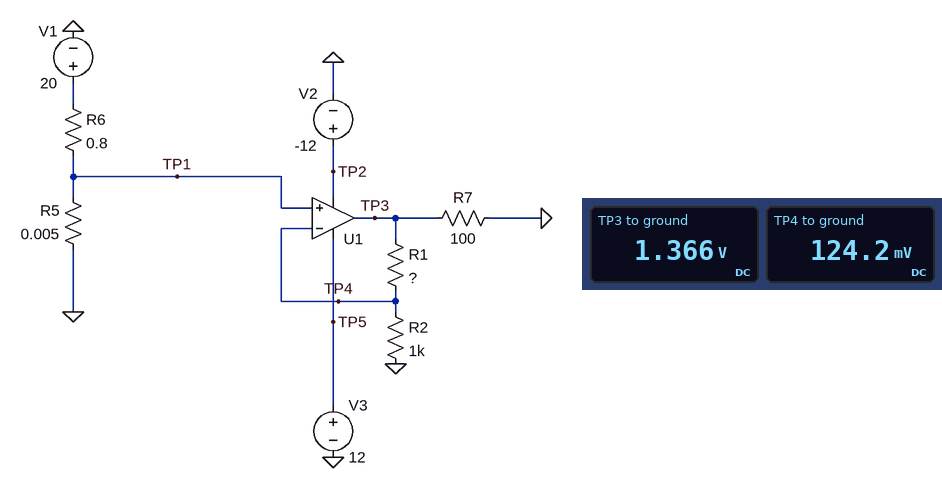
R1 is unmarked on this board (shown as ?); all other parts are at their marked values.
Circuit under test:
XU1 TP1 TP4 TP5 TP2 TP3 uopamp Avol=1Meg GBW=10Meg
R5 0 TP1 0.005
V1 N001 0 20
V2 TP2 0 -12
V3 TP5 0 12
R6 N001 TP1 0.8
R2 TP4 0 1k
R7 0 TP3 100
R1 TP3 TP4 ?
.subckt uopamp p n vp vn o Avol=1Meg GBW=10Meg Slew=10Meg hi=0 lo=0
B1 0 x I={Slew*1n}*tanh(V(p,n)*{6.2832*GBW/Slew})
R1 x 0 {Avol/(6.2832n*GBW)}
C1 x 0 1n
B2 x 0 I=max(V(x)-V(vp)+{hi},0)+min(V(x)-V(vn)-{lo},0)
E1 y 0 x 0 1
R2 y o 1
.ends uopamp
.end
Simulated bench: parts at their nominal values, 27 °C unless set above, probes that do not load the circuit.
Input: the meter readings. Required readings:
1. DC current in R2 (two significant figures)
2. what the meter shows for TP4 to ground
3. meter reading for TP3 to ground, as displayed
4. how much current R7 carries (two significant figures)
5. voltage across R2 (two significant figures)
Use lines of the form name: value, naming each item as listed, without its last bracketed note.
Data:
DC current in R2: 120 µA
what the meter shows for TP4 to ground: 124.2 mV
meter reading for TP3 to ground, as displayed: 1.366 V
how much current R7 carries: 14 mA
voltage across R2: 120 mV
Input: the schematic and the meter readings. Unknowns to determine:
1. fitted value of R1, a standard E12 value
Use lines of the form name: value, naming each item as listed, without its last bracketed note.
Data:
fitted value of R1, a standard E12 value: 10 kΩ
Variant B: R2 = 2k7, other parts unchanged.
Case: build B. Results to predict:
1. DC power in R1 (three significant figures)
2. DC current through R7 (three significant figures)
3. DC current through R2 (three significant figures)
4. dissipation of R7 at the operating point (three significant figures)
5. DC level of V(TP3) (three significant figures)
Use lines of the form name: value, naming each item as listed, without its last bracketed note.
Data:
DC power in R1: 21.2 µW
DC current through R7: 5.84 mA
DC current through R2: 46.0 µA
dissipation of R7 at the operating point: 3.41 mW
DC level of V(TP3): 584 mV
